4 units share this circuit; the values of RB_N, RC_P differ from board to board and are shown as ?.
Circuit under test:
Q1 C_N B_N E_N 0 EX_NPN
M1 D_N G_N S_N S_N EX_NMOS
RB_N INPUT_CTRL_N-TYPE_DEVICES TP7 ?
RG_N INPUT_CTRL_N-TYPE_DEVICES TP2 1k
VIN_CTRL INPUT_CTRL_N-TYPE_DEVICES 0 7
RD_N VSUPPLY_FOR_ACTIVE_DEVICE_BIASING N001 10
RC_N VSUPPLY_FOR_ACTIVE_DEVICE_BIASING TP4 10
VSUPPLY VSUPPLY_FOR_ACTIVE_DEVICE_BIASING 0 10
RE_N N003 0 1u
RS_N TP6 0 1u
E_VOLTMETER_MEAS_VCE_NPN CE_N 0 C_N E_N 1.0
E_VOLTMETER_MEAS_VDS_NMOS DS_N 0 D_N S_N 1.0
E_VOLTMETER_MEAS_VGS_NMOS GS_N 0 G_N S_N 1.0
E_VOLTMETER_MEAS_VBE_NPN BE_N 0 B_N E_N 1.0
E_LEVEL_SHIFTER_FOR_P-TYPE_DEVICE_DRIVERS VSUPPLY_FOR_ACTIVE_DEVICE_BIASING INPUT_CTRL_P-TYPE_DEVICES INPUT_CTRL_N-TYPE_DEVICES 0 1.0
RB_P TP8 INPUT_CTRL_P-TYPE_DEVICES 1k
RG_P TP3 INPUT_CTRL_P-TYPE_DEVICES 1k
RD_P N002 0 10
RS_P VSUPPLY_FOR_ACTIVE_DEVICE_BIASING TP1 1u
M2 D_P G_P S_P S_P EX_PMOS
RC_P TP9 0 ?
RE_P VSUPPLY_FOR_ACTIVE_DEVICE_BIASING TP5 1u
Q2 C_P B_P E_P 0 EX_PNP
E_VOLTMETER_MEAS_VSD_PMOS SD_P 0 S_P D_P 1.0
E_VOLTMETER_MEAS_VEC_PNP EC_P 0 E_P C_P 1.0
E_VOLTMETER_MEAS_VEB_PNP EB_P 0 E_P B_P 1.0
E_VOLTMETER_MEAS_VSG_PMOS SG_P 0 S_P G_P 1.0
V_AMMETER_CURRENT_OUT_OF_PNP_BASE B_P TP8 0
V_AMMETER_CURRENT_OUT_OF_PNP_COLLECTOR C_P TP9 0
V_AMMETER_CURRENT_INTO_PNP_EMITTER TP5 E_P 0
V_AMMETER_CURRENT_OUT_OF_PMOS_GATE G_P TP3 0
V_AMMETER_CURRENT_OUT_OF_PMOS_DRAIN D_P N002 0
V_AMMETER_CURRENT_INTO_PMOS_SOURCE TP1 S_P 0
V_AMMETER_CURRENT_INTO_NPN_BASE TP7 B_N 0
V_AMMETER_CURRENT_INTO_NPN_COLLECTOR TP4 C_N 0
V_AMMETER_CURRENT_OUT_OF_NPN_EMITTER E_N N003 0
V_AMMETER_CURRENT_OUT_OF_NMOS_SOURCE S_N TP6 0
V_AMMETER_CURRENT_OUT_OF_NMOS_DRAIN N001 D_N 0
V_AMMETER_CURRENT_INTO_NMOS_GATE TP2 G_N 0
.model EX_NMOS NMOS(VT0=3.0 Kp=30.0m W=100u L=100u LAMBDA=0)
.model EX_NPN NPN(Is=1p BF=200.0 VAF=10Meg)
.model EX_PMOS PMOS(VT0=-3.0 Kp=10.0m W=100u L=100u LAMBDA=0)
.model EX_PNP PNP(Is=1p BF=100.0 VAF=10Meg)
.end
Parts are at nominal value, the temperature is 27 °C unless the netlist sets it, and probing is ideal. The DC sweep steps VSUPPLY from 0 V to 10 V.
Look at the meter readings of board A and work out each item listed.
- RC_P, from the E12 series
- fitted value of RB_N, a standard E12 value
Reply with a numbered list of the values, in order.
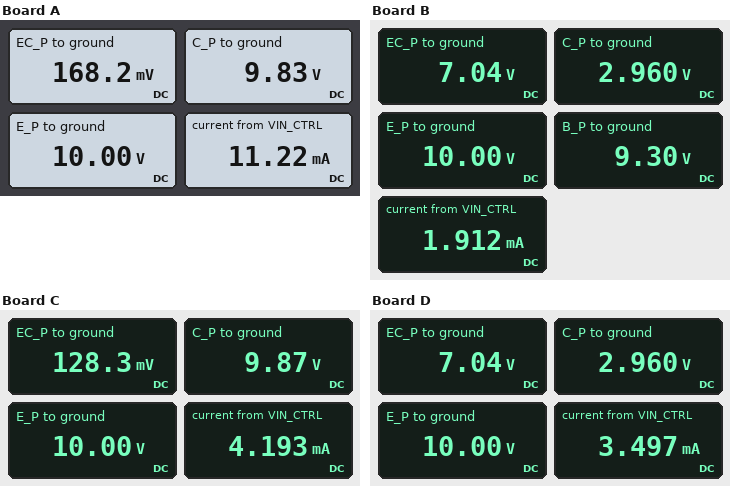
1. 18 Ω
2. 560 Ω
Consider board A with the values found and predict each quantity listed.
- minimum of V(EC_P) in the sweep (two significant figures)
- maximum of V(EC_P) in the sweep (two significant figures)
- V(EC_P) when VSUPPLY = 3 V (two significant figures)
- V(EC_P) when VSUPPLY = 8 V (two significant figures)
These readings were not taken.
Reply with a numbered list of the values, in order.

1. 16 mV
2. 170 mV
3. 93 mV
4. 140 mV
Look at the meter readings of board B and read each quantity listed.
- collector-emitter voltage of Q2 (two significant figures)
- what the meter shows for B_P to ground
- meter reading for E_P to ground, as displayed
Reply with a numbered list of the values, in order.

1. -7.0 V
2. 9.30 V
3. 10.00 V
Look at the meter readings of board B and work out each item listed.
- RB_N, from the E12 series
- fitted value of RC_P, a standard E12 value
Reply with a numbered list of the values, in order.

1. 3.3 kΩ
2. 4.7 Ω
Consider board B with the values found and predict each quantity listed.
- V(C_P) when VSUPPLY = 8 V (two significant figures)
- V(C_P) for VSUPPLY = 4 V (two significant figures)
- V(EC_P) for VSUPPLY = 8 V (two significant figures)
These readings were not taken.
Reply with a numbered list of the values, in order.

1. 3.0 V
2. 3.0 V
3. 5.0 V
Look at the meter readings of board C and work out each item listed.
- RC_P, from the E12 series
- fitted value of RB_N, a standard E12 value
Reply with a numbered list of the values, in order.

1. 27 Ω
2. 1.5 kΩ
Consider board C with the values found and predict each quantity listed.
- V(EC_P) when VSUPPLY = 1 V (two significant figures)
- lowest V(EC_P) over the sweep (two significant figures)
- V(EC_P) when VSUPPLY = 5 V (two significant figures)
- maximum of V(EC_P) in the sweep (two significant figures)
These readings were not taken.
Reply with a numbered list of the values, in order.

1. 54 mV
2. 17 mV
3. 97 mV
4. 130 mV
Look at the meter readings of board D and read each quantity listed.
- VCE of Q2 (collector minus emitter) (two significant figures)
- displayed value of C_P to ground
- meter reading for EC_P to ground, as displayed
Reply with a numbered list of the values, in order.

1. -7.0 V
2. 2.960 V
3. 7.04 V
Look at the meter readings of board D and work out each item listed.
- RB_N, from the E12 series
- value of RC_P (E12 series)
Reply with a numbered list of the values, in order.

1. 1.8 kΩ
2. 4.7 Ω
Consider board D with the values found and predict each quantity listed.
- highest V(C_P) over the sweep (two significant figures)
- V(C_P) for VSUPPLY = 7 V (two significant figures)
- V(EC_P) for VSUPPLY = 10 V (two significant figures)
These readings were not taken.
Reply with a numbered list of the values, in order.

1. 3.0 V
2. 3.0 V
3. 7.0 V
